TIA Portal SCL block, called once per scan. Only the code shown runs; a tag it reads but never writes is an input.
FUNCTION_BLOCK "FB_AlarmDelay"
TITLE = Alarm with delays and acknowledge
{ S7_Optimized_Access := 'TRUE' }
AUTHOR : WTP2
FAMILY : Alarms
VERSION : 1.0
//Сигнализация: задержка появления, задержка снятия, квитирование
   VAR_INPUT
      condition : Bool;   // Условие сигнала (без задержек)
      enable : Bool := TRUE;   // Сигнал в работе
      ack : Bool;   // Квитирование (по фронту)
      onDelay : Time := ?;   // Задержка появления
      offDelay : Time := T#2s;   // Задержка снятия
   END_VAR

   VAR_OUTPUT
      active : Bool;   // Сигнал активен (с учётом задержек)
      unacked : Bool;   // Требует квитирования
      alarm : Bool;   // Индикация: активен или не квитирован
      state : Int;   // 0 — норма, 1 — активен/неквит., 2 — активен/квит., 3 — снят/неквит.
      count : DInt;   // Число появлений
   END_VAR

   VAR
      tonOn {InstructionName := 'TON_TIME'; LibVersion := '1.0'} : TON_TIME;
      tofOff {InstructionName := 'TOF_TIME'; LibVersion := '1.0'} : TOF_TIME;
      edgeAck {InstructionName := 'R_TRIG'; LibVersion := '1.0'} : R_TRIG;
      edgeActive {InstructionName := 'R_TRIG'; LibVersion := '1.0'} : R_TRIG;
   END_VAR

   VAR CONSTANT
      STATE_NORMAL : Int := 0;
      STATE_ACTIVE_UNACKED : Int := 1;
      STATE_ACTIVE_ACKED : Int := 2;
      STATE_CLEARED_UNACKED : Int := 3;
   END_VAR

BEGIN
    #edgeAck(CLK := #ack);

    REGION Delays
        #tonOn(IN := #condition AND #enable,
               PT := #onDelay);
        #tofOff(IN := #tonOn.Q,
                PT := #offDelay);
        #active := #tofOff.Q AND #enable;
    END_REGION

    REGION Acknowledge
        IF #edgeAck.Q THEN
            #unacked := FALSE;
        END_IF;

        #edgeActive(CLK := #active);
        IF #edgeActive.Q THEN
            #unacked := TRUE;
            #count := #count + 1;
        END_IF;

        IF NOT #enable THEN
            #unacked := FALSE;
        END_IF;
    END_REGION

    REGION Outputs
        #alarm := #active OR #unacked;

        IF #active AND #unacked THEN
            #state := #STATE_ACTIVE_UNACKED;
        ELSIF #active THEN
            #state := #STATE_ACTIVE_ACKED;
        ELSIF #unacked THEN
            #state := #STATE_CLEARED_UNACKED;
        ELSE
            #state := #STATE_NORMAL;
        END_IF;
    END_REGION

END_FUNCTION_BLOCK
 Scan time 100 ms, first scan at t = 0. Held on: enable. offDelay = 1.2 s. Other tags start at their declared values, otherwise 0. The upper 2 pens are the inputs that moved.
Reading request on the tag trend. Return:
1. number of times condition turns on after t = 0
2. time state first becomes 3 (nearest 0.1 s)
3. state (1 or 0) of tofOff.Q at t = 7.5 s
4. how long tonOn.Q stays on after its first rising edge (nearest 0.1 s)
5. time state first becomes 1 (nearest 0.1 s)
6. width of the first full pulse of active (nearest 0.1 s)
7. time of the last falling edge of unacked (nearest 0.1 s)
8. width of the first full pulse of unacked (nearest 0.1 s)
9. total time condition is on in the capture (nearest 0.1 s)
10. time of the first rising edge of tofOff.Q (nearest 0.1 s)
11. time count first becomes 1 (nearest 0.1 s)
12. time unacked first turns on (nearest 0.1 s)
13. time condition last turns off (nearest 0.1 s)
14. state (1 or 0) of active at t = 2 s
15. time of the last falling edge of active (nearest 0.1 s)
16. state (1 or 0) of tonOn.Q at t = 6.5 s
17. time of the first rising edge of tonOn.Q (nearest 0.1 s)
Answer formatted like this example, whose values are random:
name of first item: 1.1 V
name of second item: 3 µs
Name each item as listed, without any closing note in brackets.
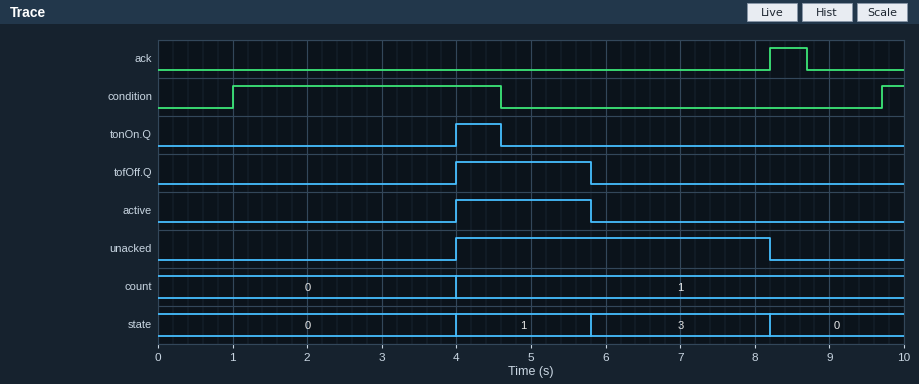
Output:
number of times condition turns on after t = 0: 2
time state first becomes 3: 5.8 s
state (1 or 0) of tofOff.Q at t = 7.5 s: 0
how long tonOn.Q stays on after its first rising edge: 0.6 s
time state first becomes 1: 4.0 s
width of the first full pulse of active: 1.8 s
time of the last falling edge of unacked: 8.2 s
width of the first full pulse of unacked: 4.2 s
total time condition is on in the capture: 3.9 s
time of the first rising edge of tofOff.Q: 4.0 s
time count first becomes 1: 4.0 s
time unacked first turns on: 4.0 s
time condition last turns off: 4.6 s
state (1 or 0) of active at t = 2 s: 0
time of the last falling edge of active: 5.8 s
state (1 or 0) of tonOn.Q at t = 6.5 s: 0
time of the first rising edge of tonOn.Q: 4.0 s
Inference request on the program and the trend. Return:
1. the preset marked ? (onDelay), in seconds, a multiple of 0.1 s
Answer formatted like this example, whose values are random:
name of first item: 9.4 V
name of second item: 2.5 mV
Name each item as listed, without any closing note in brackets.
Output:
the preset marked ? (onDelay), in seconds, a multiple of 0.1 s: 3.0 s
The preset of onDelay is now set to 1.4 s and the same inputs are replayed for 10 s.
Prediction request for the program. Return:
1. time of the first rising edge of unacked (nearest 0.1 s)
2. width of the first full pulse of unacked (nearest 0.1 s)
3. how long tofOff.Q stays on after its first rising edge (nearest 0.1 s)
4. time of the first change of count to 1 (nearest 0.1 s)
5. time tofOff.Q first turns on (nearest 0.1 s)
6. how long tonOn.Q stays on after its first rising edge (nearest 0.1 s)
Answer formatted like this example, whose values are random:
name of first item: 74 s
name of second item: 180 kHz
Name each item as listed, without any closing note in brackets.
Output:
time of the first rising edge of unacked: 2.4 s
width of the first full pulse of unacked: 5.8 s
how long tofOff.Q stays on after its first rising edge: 3.4 s
time of the first change of count to 1: 2.4 s
time tofOff.Q first turns on: 2.4 s
how long tonOn.Q stays on after its first rising edge: 2.2 s
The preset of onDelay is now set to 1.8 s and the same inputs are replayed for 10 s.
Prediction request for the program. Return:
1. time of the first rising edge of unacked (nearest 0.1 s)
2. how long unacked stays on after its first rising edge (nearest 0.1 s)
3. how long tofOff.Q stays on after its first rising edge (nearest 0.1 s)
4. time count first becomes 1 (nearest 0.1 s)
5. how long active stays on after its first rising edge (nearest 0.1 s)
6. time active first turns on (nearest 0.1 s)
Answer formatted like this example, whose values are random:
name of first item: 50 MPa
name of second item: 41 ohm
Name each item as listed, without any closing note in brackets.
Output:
time of the first rising edge of unacked: 2.8 s
how long unacked stays on after its first rising edge: 5.4 s
how long tofOff.Q stays on after its first rising edge: 3.0 s
time count first becomes 1: 2.8 s
how long active stays on after its first rising edge: 3.0 s
time active first turns on: 2.8 s
